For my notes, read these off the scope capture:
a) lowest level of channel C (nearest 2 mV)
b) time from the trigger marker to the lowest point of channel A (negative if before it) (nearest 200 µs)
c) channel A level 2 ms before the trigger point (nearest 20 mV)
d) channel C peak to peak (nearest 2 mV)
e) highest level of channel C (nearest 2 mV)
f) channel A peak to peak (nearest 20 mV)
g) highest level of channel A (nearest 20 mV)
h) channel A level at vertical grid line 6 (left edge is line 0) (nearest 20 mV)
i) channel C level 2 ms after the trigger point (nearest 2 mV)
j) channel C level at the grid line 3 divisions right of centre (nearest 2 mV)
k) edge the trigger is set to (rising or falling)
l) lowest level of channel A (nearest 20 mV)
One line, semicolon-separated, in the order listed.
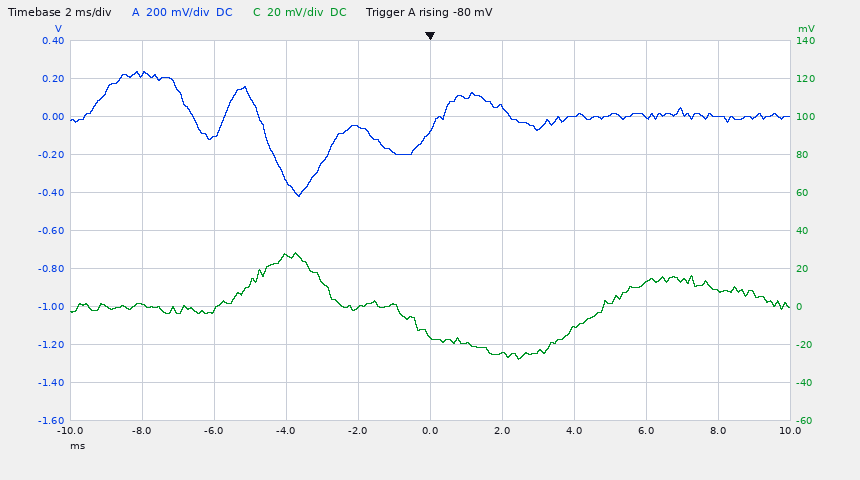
-28 mV; -3.6 ms; -60 mV; 56 mV; 28 mV; 660 mV; 240 mV; 40 mV; -24 mV; 12 mV; rising; -420 mV
